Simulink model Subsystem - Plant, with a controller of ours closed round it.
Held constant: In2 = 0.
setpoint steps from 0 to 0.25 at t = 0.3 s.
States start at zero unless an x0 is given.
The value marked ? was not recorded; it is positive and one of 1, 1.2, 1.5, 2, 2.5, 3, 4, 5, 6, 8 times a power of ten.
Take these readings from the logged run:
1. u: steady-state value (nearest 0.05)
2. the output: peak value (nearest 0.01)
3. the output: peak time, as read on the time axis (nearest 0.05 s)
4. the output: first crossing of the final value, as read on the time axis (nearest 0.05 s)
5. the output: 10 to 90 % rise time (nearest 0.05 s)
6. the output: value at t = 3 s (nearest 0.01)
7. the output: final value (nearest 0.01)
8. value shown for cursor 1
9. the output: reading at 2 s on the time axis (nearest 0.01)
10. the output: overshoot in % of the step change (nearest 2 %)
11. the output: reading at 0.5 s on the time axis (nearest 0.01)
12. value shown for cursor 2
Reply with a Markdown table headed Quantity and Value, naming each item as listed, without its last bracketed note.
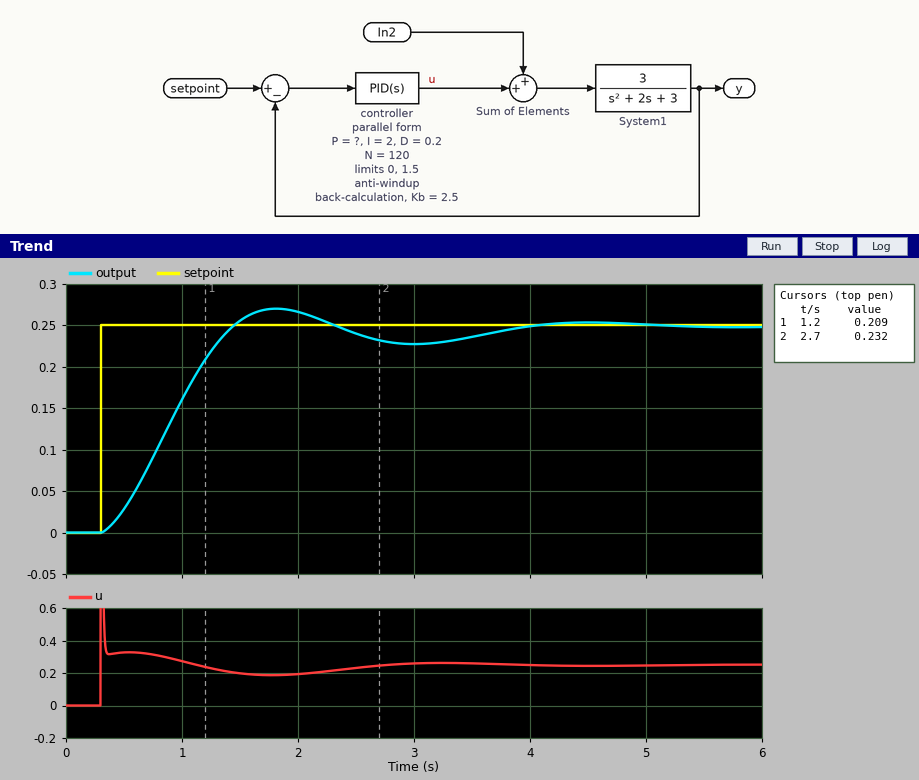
| Quantity | Value |
|---|---|
| u: steady-state value | 0.25 |
| the output: peak value | 0.27 |
| the output: peak time, as read on the time axis | 1.80 s |
| the output: first crossing of the final value, as read on the time axis | 1.45 s |
| the output: 10 to 90 % rise time | 0.80 s |
| the output: value at t = 3 s | 0.23 |
| the output: final value | 0.25 |
| value shown for cursor 1 | 0.209 |
| the output: reading at 2 s on the time axis | 0.27 |
| the output: overshoot in % of the step change | 8 % |
| the output: reading at 0.5 s on the time axis | 0.03 |
| value shown for cursor 2 | 0.232 |
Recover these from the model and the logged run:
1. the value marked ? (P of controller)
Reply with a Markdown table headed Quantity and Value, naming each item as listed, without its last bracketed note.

| Quantity | Value |
|---|---|
| the value marked ? | 1.5 |
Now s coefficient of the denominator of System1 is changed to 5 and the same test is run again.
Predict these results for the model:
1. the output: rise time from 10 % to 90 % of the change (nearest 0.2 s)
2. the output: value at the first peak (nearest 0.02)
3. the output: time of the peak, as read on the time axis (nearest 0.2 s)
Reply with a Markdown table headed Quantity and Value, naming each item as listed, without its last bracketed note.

| Quantity | Value |
|---|---|
| the output: rise time from 10 % to 90 % of the change | 1.2 s |
| the output: value at the first peak | 0.28 |
| the output: time of the peak, as read on the time axis | 3.0 s |
